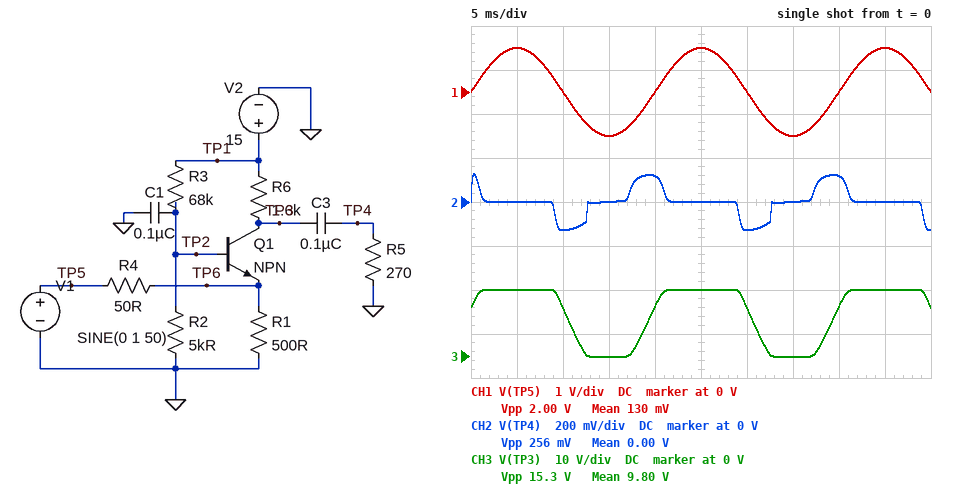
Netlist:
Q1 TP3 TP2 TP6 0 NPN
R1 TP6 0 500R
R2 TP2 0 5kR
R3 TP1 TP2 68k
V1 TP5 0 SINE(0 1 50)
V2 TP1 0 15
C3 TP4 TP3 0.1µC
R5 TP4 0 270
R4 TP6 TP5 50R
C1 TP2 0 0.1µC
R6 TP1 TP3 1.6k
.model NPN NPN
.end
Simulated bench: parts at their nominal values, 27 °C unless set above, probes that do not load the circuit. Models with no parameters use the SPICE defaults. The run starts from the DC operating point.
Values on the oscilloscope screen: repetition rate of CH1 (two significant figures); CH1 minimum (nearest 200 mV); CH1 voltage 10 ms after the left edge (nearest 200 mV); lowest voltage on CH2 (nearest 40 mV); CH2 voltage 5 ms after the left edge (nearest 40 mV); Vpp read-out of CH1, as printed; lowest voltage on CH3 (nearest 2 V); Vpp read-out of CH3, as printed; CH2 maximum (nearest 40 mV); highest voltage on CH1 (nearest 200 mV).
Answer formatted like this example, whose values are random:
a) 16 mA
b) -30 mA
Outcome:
a) 50 Hz
b) -1.0 V
c) 0 V
d) -120 mV
e) 0 V
f) 2.00 V
g) 0 V
h) 15.3 V
i) 120 mV
j) 1.0 V
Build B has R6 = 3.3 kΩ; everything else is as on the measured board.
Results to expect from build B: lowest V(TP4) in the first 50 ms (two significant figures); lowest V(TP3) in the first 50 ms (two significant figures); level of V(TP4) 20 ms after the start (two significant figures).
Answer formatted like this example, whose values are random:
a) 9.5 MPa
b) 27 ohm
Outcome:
a) -260 mV
b) -590 mV
c) 220 mV
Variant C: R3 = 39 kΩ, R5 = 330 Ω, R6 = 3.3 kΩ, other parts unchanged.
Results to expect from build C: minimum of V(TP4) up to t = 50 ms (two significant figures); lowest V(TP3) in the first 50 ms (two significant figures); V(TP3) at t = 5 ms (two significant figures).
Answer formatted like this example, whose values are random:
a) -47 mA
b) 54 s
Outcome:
a) -270 mV
b) -600 mV
c) 13 V
